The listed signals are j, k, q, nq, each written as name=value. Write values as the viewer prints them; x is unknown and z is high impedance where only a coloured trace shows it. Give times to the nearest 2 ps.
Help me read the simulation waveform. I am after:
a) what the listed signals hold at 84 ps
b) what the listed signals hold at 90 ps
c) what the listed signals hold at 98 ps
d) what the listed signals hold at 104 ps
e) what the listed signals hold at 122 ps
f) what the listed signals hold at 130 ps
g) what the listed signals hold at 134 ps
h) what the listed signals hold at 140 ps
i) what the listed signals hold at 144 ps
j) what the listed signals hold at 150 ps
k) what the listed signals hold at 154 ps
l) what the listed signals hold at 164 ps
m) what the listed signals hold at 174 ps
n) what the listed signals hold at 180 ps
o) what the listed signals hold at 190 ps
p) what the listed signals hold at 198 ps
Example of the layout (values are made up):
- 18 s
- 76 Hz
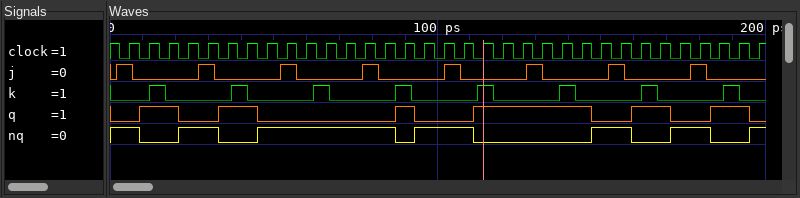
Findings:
- j=0, k=0, q=0, nq=1
- j=0, k=1, q=1, nq=0
- j=0, k=0, q=0, nq=1
- j=1, k=0, q=0, nq=1
- j=0, k=0, q=1, nq=0
- j=1, k=0, q=1, nq=0
- j=0, k=0, q=1, nq=0
- j=0, k=1, q=1, nq=0
- j=0, k=0, q=1, nq=0
- j=0, k=0, q=0, nq=1
- j=1, k=0, q=0, nq=1
- j=0, k=1, q=1, nq=0
- j=0, k=0, q=0, nq=1
- j=1, k=0, q=0, nq=1
- j=0, k=1, q=1, nq=0
- j=0, k=0, q=0, nq=1
